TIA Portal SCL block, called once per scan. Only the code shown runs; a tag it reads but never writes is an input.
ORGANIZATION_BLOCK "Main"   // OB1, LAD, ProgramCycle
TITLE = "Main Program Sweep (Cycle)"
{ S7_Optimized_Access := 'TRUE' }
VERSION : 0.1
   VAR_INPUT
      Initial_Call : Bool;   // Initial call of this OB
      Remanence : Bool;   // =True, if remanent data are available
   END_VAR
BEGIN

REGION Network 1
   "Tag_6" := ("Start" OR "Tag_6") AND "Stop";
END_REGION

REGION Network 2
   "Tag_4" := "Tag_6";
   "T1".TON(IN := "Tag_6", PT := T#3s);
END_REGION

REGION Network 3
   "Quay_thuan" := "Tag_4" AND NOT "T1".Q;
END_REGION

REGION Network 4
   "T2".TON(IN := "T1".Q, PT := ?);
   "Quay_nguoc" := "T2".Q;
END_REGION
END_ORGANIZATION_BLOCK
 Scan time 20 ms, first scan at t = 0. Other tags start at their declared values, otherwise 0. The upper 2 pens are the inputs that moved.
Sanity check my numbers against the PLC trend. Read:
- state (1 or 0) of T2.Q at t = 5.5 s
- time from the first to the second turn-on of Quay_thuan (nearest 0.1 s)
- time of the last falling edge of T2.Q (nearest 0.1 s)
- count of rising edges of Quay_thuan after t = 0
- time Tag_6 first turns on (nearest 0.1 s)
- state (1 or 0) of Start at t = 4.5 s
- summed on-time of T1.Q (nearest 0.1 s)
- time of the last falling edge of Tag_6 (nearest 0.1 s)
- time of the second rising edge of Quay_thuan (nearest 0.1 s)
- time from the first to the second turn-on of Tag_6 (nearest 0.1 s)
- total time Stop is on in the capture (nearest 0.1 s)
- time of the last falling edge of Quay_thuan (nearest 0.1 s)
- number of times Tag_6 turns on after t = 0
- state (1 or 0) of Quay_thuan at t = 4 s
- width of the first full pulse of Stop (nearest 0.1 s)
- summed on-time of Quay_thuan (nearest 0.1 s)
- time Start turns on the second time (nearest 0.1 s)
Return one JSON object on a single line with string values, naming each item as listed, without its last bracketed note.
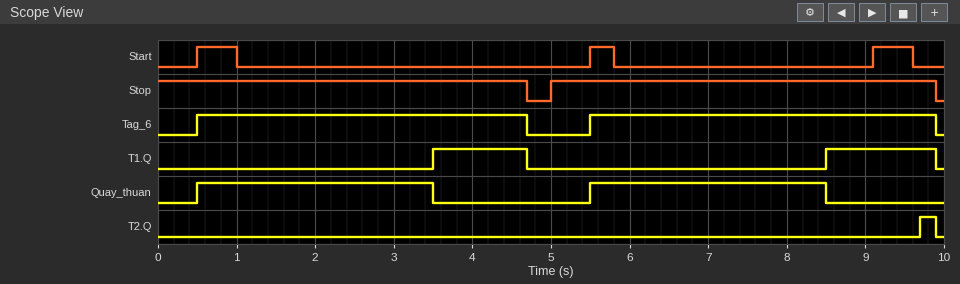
{"state (1 or 0) of T2.Q at t = 5.5 s": "0", "time from the first to the second turn-on of Quay_thuan": "5.0 s", "time of the last falling edge of T2.Q": "9.9 s", "count of rising edges of Quay_thuan after t = 0": "2", "time Tag_6 first turns on": "0.5 s", "state (1 or 0) of Start at t = 4.5 s": "0", "summed on-time of T1.Q": "2.6 s", "time of the last falling edge of Tag_6": "9.9 s", "time of the second rising edge of Quay_thuan": "5.5 s", "time from the first to the second turn-on of Tag_6": "5.0 s", "total time Stop is on in the capture": "9.6 s", "time of the last falling edge of Quay_thuan": "8.5 s", "number of times Tag_6 turns on after t = 0": "2", "state (1 or 0) of Quay_thuan at t = 4 s": "0", "width of the first full pulse of Stop": "4.9 s", "summed on-time of Quay_thuan": "6.0 s", "time Start turns on the second time": "5.5 s"}
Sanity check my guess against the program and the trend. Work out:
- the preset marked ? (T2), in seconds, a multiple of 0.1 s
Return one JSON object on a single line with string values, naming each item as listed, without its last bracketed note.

{"the preset marked ? (T2), in seconds, a multiple of 0.1 s": "1.2 s"}
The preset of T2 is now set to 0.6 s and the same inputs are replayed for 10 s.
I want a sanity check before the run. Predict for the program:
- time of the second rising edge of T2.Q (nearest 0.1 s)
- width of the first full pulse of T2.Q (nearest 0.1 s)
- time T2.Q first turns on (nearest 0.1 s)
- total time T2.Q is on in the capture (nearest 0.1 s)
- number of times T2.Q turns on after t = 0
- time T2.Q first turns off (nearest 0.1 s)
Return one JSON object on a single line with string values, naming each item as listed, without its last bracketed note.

{"time of the second rising edge of T2.Q": "9.1 s", "width of the first full pulse of T2.Q": "0.6 s", "time T2.Q first turns on": "4.1 s", "total time T2.Q is on in the capture": "1.4 s", "number of times T2.Q turns on after t = 0": "2", "time T2.Q first turns off": "4.7 s"}
